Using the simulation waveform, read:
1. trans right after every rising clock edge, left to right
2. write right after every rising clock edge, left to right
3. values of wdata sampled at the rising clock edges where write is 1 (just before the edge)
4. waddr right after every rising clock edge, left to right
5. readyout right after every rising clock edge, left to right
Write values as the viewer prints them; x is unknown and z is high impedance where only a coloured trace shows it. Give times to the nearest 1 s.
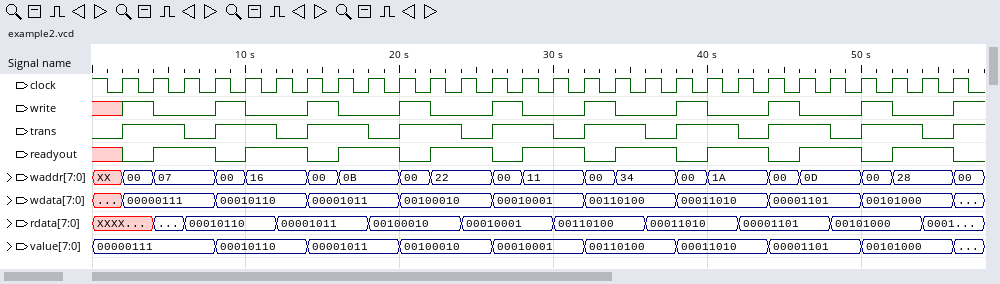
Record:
1 1 0 1 1 0 1 1 0 1 1 0 1 1 0 1 1 0 1 1 0 1 1 0 1 1 0 1
1 0 0 1 0 0 1 0 0 1 0 0 1 0 0 1 0 0 1 0 0 1 0 0 1 0 0 1
00000111, 00010110, 00001011, 00100010, 00010001, 00110100, 00011010, 00001101, 00101000
00, 07, 07, 00, 16, 16, 00, 0B, 0B, 00, 22, 22, 00, 11, 11, 00, 34, 34, 00, 1A, 1A, 00, 0D, 0D, 00, 28, 28, 00
0 1 1 0 1 1 0 1 1 0 1 1 0 1 1 0 1 1 0 1 1 0 1 1 0 1 1 0
